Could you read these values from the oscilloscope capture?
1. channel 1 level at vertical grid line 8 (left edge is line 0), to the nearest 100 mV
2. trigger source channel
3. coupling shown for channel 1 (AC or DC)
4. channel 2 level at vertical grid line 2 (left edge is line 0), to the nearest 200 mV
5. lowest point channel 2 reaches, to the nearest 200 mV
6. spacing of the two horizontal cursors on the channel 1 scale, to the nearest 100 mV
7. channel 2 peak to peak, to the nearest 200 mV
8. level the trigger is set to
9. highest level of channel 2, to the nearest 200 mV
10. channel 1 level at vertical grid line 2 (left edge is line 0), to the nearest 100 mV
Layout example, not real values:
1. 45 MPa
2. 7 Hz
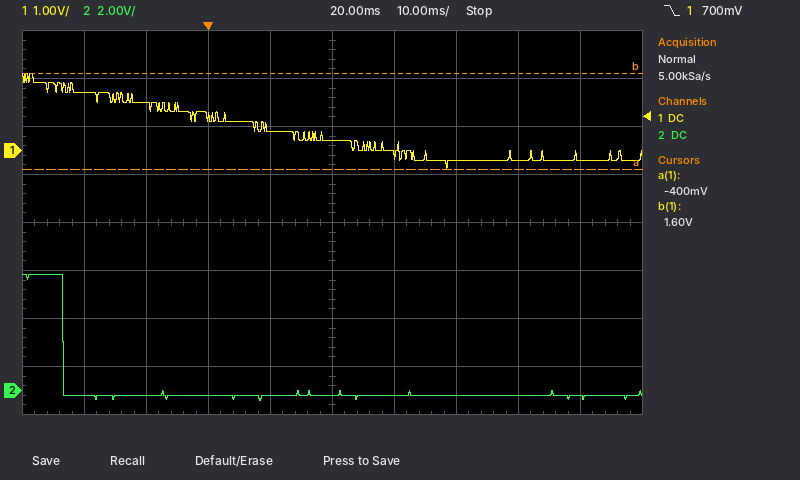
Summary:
1. -200 mV
2. channel 1
3. DC
4. -200 mV
5. -400 mV
6. 2.0 V
7. 5.2 V
8. 700 mV
9. 4.8 V
10. 1.0 V
